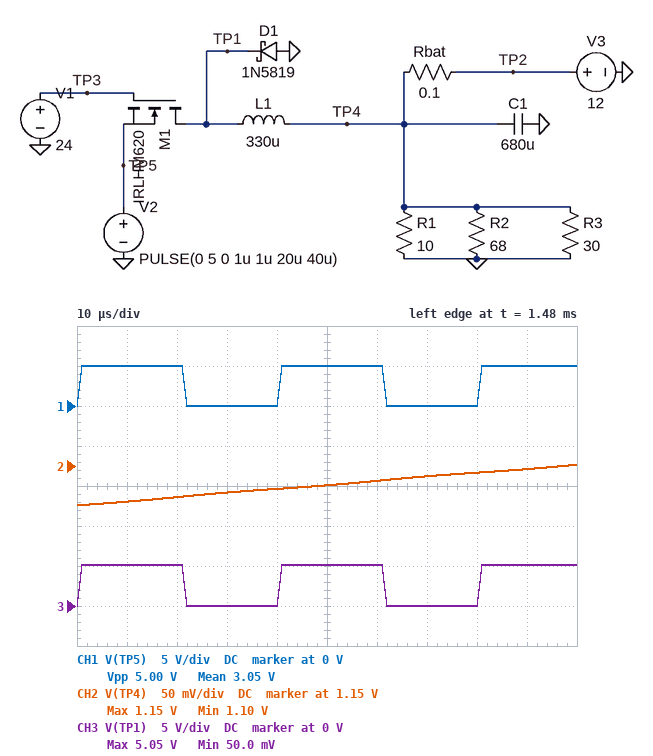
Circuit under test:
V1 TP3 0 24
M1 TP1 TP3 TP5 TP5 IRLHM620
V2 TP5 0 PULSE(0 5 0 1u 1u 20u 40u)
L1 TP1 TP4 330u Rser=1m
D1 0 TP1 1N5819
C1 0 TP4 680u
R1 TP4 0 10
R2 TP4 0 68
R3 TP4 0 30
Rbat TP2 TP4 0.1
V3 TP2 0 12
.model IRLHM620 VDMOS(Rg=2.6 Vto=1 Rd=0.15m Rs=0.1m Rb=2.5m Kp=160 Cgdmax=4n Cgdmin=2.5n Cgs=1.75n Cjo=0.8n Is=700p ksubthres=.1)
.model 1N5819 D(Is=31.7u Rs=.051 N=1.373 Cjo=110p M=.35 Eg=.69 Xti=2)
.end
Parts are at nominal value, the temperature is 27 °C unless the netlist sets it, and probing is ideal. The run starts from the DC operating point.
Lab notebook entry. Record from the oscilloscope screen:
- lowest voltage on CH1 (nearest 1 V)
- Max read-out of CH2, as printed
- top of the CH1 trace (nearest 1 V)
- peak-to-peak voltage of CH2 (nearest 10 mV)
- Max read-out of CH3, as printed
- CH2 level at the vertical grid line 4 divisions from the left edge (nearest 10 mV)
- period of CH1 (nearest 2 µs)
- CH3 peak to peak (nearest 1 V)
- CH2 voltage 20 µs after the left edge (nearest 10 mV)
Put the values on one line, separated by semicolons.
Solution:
0 V; 1.15 V; 5 V; 50 mV; 5.05 V; 1.12 V; 40 µs; 5 V; 1.11 V
